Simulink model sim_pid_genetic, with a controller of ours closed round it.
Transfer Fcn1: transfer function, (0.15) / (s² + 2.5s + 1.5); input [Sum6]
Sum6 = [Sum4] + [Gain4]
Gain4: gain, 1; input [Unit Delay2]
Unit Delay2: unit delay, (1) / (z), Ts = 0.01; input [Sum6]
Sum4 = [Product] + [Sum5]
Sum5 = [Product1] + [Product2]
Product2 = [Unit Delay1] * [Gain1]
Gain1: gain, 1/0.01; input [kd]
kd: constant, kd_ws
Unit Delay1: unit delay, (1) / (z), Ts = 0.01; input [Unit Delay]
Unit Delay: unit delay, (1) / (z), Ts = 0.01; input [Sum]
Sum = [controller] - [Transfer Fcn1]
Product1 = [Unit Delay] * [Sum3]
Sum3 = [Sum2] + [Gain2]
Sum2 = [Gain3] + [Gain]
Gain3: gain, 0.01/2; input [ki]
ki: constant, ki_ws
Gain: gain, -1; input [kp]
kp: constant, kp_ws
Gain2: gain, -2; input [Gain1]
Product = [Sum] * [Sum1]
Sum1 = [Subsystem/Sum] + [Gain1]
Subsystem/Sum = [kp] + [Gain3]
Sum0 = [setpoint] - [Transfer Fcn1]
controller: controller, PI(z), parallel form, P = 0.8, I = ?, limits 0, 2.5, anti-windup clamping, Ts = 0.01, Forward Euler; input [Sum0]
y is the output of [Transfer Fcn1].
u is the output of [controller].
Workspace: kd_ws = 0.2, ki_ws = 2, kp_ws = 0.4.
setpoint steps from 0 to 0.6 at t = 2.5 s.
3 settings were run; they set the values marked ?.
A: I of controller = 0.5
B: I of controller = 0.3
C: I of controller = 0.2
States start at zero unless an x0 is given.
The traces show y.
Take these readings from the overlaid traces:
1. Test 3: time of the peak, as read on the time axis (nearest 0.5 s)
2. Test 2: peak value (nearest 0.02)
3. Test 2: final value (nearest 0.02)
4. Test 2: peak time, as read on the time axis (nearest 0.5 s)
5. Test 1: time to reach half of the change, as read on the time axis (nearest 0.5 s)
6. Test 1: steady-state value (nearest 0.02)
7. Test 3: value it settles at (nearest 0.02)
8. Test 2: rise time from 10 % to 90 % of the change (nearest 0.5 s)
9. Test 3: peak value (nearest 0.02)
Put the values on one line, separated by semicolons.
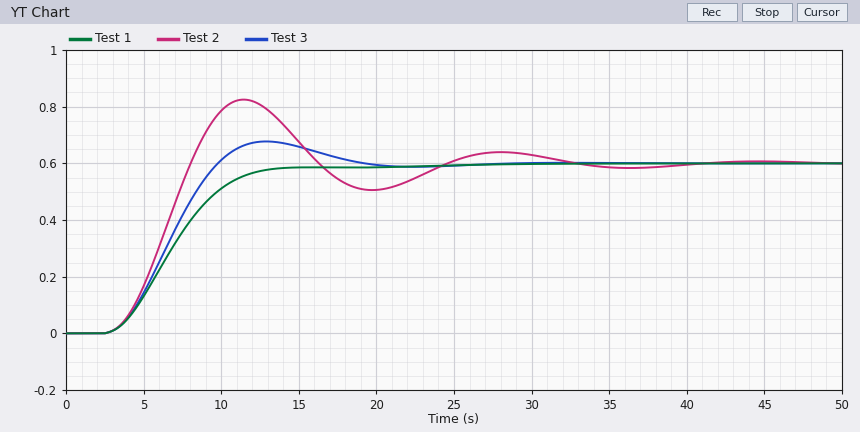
13.0 s; 0.82; 0.60; 11.5 s; 7.0 s; 0.60; 0.60; 3.5 s; 0.68
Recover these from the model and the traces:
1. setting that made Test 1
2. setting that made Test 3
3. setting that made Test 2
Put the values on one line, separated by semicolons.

C; B; A
